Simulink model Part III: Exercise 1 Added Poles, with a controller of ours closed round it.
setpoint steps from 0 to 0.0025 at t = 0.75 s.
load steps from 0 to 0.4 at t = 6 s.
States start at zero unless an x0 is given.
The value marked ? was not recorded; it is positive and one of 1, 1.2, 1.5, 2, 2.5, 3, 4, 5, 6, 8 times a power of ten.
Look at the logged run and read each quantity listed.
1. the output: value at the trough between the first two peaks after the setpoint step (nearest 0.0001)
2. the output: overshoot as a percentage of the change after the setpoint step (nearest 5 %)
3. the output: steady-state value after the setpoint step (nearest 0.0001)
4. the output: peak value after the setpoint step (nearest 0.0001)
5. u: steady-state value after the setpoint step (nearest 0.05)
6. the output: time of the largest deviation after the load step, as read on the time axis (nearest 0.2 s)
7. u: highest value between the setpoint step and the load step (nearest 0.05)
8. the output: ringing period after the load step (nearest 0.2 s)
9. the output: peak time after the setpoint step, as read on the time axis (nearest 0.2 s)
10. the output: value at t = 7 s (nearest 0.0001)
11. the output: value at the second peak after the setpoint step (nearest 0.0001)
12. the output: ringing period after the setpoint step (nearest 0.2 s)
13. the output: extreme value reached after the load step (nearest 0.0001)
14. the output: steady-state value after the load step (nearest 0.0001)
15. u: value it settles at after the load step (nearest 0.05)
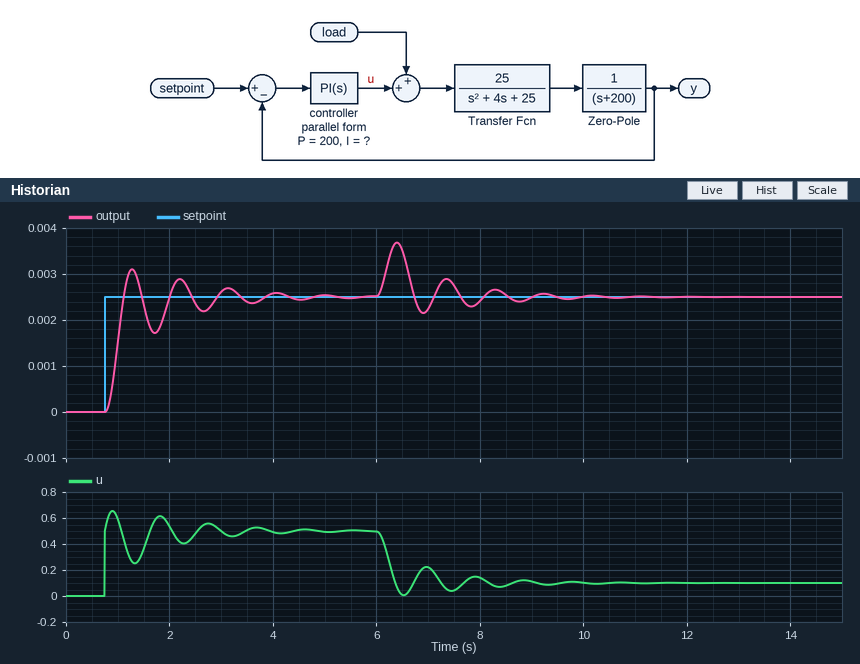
0.0017
25 %
0.0025
0.0031
0.50
6.4 s
0.65
1.0 s
1.2 s
0.0022
0.0029
1.0 s
0.0037
0.0025
0.10
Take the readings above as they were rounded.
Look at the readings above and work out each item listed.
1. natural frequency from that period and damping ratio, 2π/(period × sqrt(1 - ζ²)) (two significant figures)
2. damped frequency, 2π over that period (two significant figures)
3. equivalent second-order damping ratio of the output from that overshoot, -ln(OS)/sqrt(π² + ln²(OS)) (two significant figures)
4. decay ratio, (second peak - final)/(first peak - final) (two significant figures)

6.9 rad/s
6.3 rad/s
0.40
0.67
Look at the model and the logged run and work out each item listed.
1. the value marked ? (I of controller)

800
